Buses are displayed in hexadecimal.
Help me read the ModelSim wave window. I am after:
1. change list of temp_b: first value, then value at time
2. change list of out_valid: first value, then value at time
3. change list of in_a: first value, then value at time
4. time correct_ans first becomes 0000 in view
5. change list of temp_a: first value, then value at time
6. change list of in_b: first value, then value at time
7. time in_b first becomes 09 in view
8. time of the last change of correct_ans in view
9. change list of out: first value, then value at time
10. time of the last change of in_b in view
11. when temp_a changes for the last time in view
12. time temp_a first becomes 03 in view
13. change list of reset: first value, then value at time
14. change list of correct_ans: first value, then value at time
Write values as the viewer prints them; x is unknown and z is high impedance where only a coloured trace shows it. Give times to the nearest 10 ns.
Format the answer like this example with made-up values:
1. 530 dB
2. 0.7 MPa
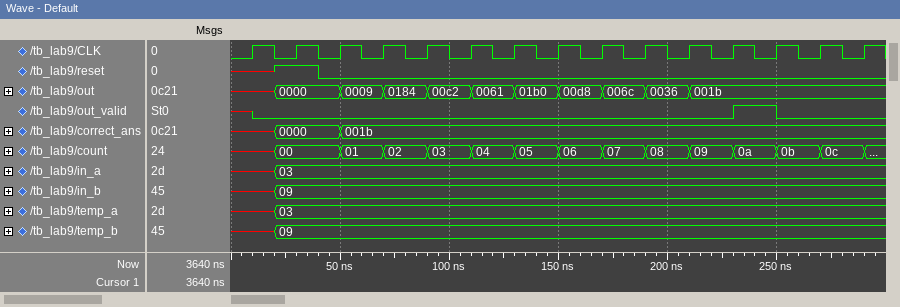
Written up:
1. x, 09 at 20 ns
2. x, 0 at 10 ns, 1 at 230 ns, 0 at 250 ns
3. x, 03 at 20 ns
4. 20 ns
5. x, 03 at 20 ns
6. x, 09 at 20 ns
7. 20 ns
8. 50 ns
9. x, 0000 at 20 ns, 0009 at 50 ns, 0184 at 70 ns, 00c2 at 90 ns, 0061 at 110 ns, 01b0 at 130 ns, 00d8 at 150 ns, 006c at 170 ns, 0036 at 190 ns, 001b at 210 ns
10. 20 ns
11. 20 ns
12. 20 ns
13. x, 1 at 20 ns, 0 at 40 ns
14. x, 0000 at 20 ns, 001b at 50 ns
